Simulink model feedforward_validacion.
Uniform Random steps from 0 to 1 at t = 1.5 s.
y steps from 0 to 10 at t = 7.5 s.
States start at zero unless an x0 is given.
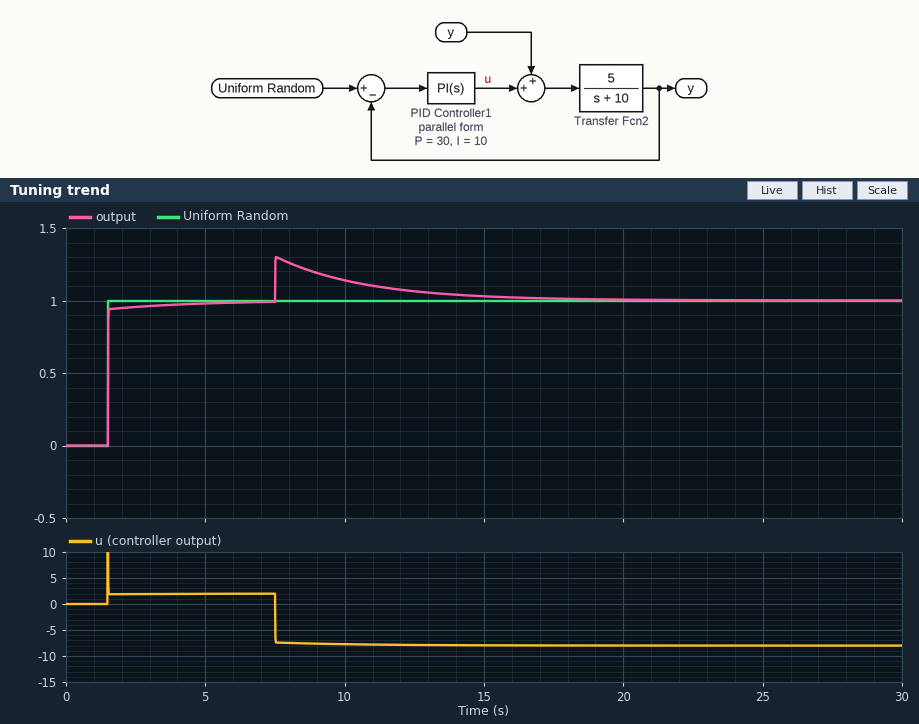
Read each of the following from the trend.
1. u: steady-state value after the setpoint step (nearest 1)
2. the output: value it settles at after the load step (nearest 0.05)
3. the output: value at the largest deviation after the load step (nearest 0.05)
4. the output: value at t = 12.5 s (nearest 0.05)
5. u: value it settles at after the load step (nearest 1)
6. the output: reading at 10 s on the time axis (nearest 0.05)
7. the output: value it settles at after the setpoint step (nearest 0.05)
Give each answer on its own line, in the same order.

2
1.00
1.30
1.05
-8
1.15
1.00
